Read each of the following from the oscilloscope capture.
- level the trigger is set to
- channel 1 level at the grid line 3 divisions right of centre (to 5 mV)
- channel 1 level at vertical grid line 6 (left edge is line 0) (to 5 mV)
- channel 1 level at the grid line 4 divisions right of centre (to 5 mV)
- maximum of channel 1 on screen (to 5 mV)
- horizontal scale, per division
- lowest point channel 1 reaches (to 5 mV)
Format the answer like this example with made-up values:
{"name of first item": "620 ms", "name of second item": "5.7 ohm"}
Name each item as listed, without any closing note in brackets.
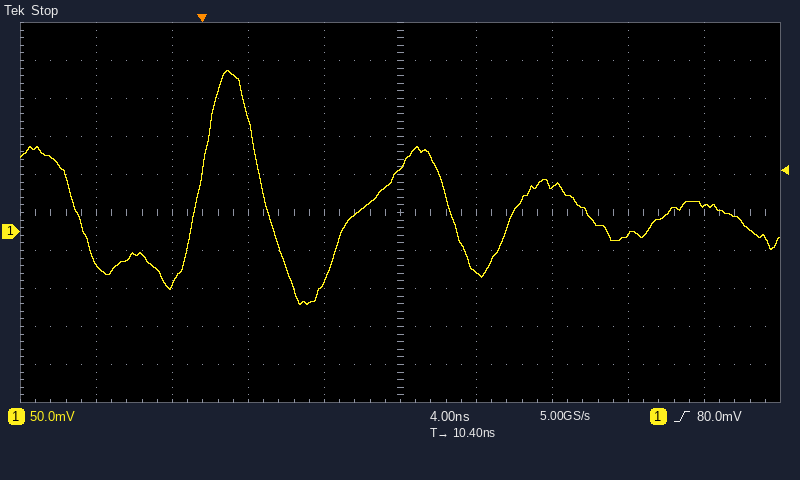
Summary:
{"level the trigger is set to": "80.0 mV", "channel 1 level at the grid line 3 divisions right of centre": "-5 mV", "channel 1 level at vertical grid line 6 (left edge is line 0)": "-55 mV", "channel 1 level at the grid line 4 divisions right of centre": "35 mV", "maximum of channel 1 on screen": "210 mV", "horizontal scale, per division": "4 ns", "lowest point channel 1 reaches": "-95 mV"}
